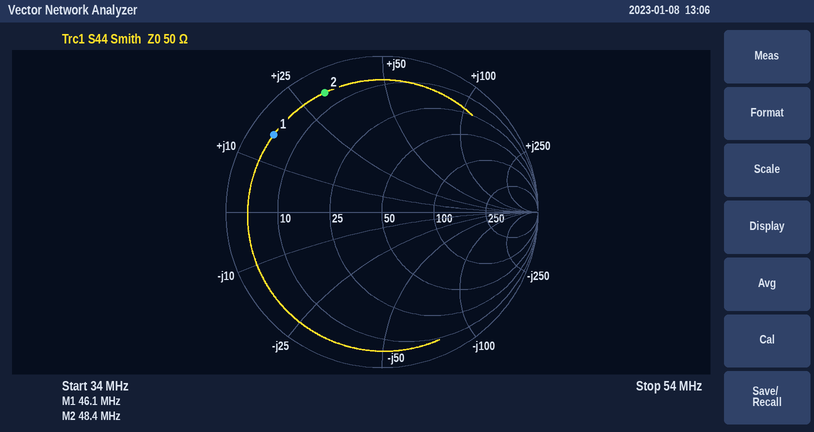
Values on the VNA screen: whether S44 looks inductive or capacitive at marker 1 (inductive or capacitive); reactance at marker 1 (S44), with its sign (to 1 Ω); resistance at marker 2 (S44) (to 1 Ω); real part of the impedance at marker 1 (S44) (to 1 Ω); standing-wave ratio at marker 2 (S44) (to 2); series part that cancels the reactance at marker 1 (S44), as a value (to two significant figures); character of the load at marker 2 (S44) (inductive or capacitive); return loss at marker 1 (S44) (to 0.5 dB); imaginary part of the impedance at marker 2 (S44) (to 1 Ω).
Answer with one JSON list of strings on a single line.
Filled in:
["inductive", "+16 Ω", "6 Ω", "4 Ω", "12", "220 pF", "inductive", "1.5 dB", "+31 Ω"]
